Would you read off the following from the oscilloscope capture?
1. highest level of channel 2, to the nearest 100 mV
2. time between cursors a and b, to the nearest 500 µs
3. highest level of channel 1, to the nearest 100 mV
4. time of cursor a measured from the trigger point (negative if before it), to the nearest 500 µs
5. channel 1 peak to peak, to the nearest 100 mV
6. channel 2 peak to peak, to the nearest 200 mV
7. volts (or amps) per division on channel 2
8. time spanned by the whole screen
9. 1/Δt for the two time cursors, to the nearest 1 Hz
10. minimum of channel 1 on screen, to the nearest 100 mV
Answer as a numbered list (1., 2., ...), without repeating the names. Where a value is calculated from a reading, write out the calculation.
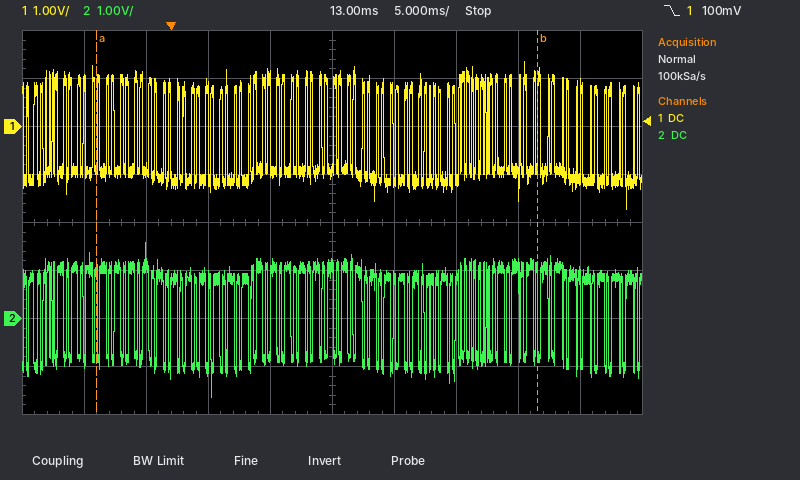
1. 1.6 V
2. 35.5 ms
3. 1.4 V
4. -6.0 ms
5. 1.4 V − (-1.7 V) = 3.1 V
6. 3.2 V
7. 1 V
8. 50 ms
9. 1 / 35.5 ms ≈ 28 Hz
10. -1.7 V
